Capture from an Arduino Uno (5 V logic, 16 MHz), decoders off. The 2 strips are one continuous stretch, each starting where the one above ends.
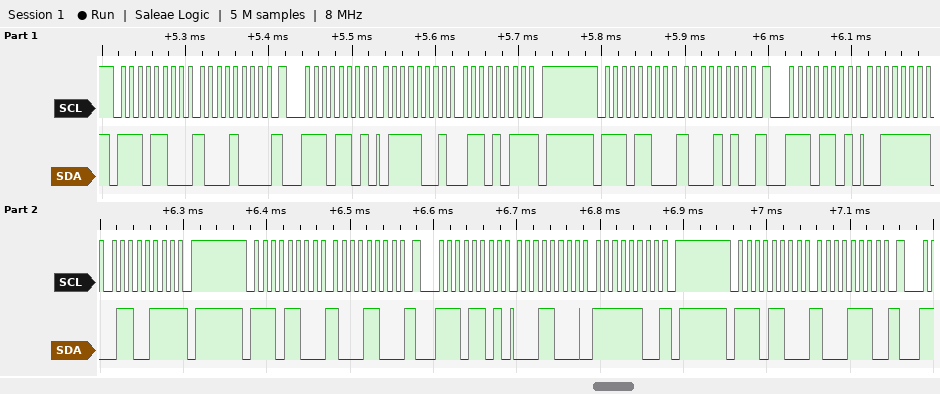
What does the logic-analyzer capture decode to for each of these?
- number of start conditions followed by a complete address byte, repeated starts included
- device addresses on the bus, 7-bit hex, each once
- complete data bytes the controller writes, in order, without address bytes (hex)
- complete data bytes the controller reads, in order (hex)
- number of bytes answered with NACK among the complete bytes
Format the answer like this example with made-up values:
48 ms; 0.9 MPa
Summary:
7; 0x76; 88 8A 8C 8E; 79 6B 3F 67 18 FC; 3
